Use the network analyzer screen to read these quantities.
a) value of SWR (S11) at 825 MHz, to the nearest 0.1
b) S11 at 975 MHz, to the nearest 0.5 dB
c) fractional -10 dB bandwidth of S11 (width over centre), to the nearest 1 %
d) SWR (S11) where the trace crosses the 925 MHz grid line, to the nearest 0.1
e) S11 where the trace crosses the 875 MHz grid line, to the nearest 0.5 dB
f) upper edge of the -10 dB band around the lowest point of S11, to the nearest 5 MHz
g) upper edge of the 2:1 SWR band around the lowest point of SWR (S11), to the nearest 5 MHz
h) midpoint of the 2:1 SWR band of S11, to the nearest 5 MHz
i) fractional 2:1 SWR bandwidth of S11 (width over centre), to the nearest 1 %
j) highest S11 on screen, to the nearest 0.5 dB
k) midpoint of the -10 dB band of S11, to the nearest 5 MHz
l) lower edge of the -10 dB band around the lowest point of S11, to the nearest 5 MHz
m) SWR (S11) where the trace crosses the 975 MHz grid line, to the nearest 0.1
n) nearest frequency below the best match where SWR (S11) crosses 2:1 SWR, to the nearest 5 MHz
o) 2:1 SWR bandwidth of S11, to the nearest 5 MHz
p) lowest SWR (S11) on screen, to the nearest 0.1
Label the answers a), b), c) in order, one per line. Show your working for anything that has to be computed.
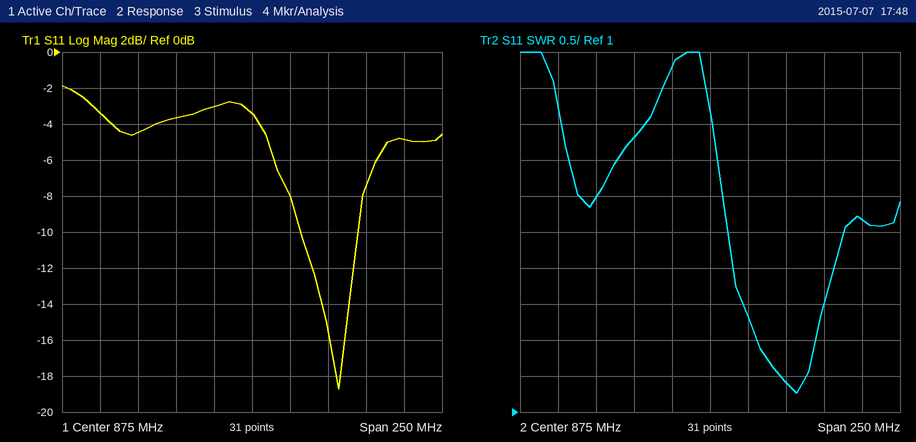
a) 4.8
b) -5.0 dB
c) 40 MHz / 925 MHz ≈ 4 %
d) 1.4
e) -3.5 dB
f) 945 MHz
g) 945 MHz
h) 925 MHz
i) 40 MHz / 925 MHz ≈ 4 %
j) -2.0 dB
k) 925 MHz
l) 905 MHz
m) 3.7
n) 905 MHz
o) 945 MHz − 905 MHz = 40 MHz
p) 1.3
